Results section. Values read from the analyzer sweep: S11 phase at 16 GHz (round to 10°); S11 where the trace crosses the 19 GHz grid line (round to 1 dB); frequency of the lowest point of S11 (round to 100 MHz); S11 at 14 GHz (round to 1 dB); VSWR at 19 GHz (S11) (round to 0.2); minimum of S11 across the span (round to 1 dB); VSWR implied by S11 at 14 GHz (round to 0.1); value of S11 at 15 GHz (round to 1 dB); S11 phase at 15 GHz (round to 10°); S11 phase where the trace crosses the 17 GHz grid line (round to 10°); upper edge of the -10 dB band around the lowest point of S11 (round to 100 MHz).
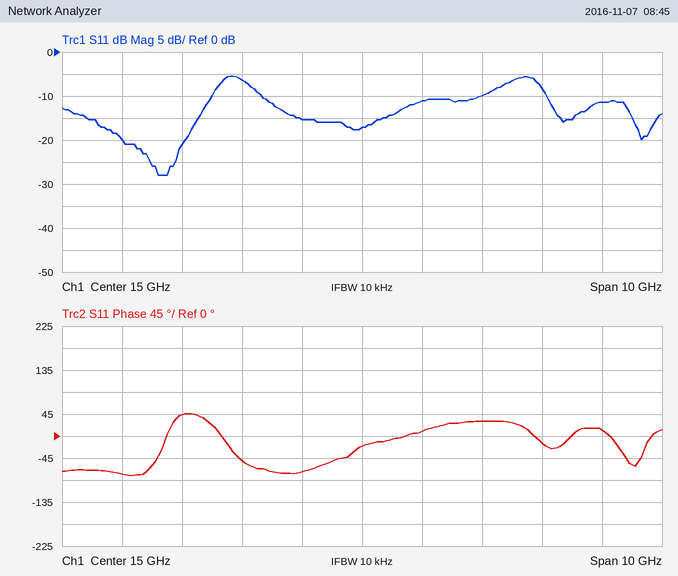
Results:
10°
-11 dB
11.6 GHz
-15 dB
1.8
-28 dB
1.4
-17 dB
-20°
30°
12.5 GHz
